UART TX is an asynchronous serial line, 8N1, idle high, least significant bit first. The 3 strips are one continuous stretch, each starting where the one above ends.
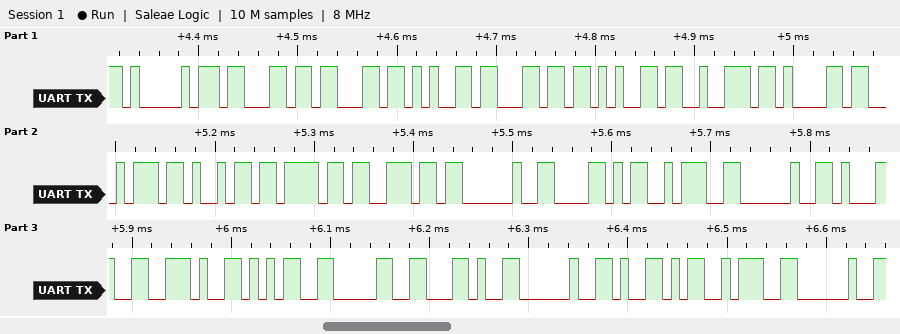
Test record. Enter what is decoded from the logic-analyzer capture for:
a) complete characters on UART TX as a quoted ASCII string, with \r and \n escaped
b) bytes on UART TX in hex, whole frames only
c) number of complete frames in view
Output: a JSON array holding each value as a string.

["\"Acceleration X: 1.50, Y: \"", "41 63 63 65 6C 65 72 61 74 69 6F 6E 20 58 3A 20 31 2E 35 30 2C 20 59 3A 20", "25"]
